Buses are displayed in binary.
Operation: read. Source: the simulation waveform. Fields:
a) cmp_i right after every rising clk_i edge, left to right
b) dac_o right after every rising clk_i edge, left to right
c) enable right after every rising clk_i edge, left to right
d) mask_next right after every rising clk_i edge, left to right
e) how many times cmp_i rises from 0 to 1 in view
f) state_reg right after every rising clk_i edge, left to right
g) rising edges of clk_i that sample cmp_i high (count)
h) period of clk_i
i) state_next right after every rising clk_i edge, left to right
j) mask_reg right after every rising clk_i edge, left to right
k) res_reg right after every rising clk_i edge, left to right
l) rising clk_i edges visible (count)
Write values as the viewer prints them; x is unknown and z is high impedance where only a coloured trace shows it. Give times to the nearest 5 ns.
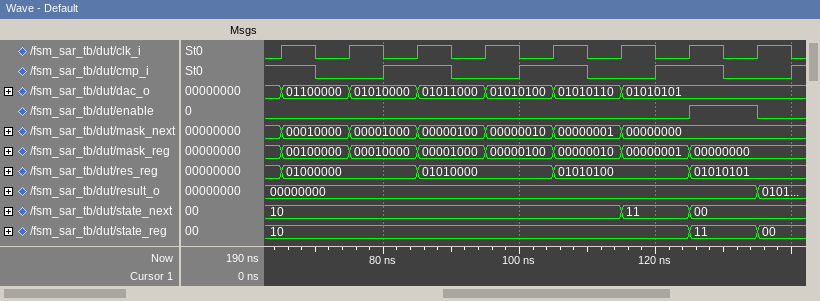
1 0 1 0 1 0 1 0
01100000, 01010000, 01011000, 01010100, 01010110, 01010101, 01010101, 01010101
0 0 0 0 0 0 1 0
00010000, 00001000, 00000100, 00000010, 00000001, 00000000, 00000000, 00000000
4
10, 10, 10, 10, 10, 10, 11, 00
4
10 ns
10, 10, 10, 10, 10, 11, 00, 00
00100000, 00010000, 00001000, 00000100, 00000010, 00000001, 00000000, 00000000
01000000, 01000000, 01010000, 01010000, 01010100, 01010100, 01010101, 01010101
8
